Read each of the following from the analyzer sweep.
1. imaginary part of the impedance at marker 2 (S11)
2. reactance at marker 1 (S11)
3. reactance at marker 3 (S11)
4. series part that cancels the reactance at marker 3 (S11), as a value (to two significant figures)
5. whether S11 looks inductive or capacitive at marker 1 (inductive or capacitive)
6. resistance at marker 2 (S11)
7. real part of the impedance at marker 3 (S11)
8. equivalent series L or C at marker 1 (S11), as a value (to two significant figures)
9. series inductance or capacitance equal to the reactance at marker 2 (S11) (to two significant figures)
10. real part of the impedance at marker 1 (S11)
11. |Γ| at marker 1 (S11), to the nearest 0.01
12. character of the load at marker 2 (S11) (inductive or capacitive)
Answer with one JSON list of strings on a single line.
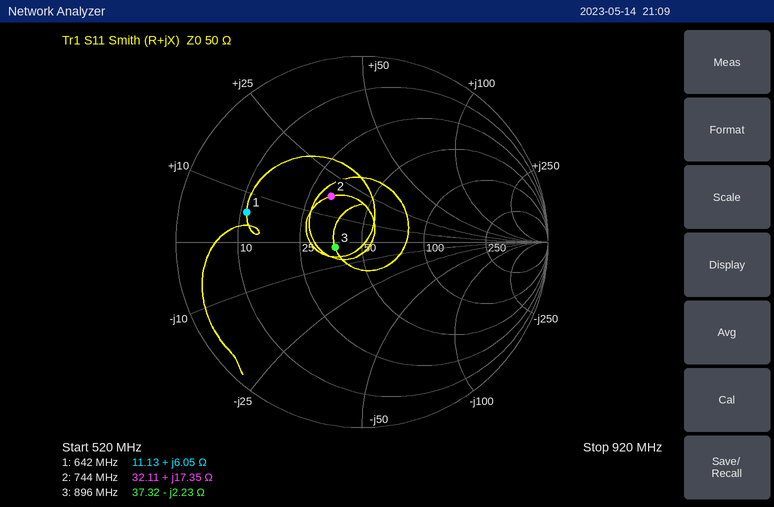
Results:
["+17.35 Ω", "+6.05 Ω", "-2.23 Ω", "400 pH", "inductive", "32.11 Ω", "37.32 Ω", "1.5 nH", "3.7 nH", "11.13 Ω", "0.64", "inductive"]
